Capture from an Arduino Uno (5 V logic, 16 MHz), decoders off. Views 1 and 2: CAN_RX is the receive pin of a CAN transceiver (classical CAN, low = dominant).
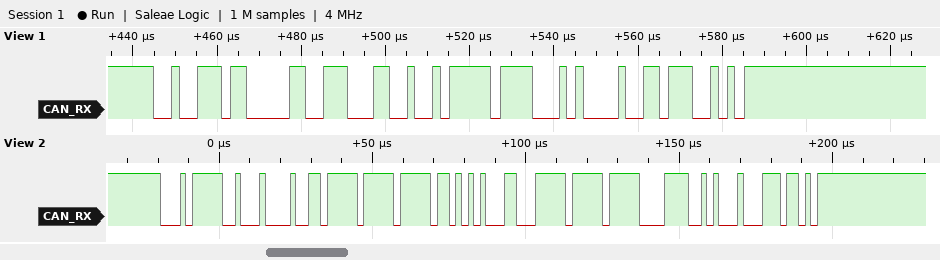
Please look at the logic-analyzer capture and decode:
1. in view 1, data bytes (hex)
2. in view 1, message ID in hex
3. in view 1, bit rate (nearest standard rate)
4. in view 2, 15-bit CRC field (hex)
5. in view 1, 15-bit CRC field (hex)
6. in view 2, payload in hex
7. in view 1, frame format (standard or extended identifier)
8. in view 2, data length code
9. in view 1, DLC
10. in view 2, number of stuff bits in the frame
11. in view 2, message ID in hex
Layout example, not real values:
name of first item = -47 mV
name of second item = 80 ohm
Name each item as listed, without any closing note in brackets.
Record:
in view 1, data bytes = E3 25 FF 14
in view 1, message ID in hex = 0x276
in view 1, bit rate = 500 kbit/s
in view 2, 15-bit CRC field = 0x4476
in view 1, 15-bit CRC field = 0x1372
in view 2, payload in hex = 4D FF FF 54 63 FF F8 F2
in view 1, frame format = standard
in view 2, data length code = 8
in view 1, DLC = 4
in view 2, number of stuff bits in the frame = 7
in view 2, message ID in hex = 0x17D
